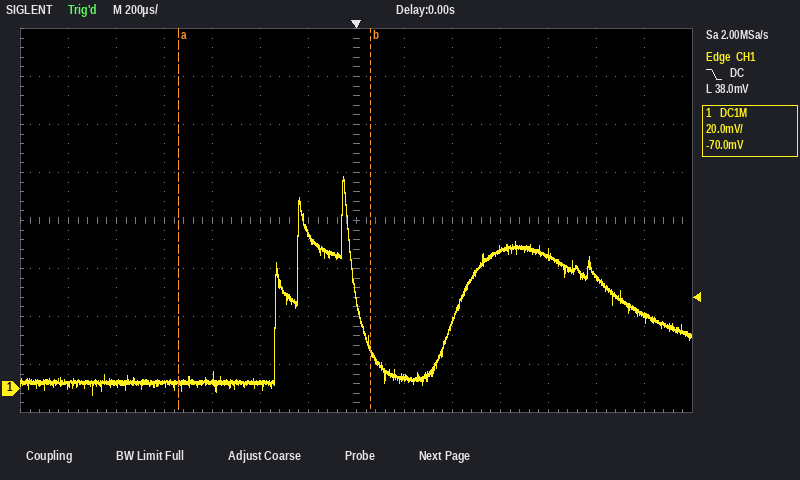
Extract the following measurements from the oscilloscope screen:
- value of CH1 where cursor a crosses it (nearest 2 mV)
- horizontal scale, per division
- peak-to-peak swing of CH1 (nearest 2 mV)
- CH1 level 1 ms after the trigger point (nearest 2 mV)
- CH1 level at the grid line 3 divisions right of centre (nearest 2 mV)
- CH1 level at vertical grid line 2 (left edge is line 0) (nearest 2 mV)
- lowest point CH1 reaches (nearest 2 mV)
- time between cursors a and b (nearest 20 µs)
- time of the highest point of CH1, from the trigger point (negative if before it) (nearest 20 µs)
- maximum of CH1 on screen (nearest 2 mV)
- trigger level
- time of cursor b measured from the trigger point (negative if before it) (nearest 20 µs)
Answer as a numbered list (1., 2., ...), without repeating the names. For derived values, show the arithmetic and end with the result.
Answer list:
1. 2 mV
2. 200 µs
3. 88 mV − (-2 mV) = 90 mV
4. 46 mV
5. 58 mV
6. 2 mV
7. -2 mV
8. 800 µs
9. -60 µs
10. 88 mV
11. 38.0 mV
12. +60 µs
